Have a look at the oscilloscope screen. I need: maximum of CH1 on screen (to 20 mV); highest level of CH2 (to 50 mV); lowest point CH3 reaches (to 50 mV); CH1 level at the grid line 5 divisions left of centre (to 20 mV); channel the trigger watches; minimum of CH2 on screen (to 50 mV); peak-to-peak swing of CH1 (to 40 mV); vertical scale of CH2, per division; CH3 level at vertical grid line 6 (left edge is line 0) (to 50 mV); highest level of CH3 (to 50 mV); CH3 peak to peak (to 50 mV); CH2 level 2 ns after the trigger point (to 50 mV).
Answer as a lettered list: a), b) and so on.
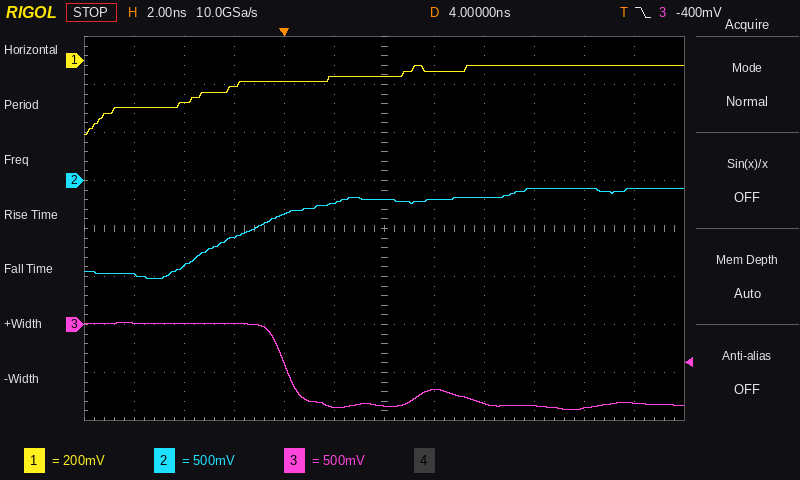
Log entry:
a) -20 mV
b) -100 mV
c) -900 mV
d) -200 mV
e) CH3
f) -1.00 V
g) 280 mV
h) 500 mV
i) -850 mV
j) 0 mV
k) 900 mV
l) -250 mV
